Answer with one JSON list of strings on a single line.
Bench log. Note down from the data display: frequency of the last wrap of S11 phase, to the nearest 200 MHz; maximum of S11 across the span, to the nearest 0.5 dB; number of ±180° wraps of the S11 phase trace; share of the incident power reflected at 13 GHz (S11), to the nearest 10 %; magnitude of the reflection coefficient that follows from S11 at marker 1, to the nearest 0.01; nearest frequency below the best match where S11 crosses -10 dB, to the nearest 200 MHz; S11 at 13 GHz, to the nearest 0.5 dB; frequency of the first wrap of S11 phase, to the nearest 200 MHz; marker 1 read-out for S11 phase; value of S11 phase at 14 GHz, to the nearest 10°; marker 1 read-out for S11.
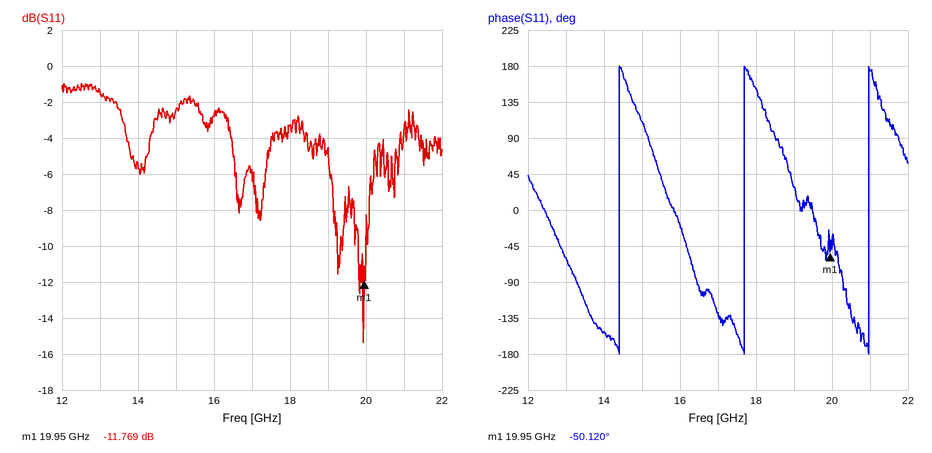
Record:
["21.0 GHz", "-1.0 dB", "3", "70 %", "0.26", "19.8 GHz", "-1.5 dB", "14.4 GHz", "-50.120°", "-150°", "-11.769 dB"]
